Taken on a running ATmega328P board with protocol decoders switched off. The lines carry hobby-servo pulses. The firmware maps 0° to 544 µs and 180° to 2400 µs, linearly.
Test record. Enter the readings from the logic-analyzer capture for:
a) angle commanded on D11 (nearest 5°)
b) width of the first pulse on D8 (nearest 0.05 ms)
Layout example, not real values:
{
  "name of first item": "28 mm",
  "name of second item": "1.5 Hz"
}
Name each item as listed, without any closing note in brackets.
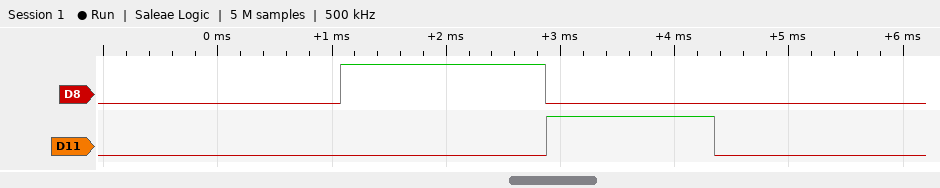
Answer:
{
  "angle commanded on D11": "90°",
  "width of the first pulse on D8": "1.80 ms"
}
